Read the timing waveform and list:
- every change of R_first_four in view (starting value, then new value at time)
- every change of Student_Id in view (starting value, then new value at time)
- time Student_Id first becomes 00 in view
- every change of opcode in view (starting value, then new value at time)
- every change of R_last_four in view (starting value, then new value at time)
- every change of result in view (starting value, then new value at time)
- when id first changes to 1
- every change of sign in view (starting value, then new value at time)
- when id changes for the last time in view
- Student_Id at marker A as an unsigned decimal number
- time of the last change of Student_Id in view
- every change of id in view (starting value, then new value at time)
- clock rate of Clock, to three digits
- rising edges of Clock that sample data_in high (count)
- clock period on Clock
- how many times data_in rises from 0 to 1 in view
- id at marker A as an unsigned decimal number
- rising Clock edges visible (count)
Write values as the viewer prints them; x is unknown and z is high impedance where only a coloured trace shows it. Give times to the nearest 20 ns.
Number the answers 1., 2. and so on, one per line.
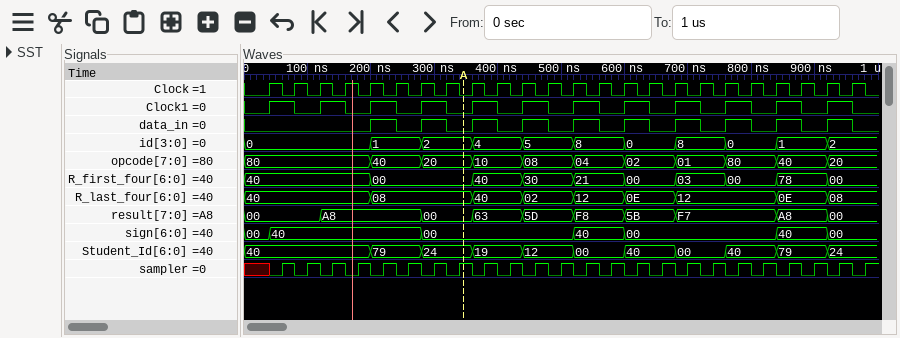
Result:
1. 40, 00 at 200 ns, 40 at 360 ns, 30 at 440 ns, 21 at 520 ns, 00 at 600 ns, 03 at 680 ns, 00 at 760 ns, 78 at 840 ns, 00 at 920 ns
2. 40, 79 at 200 ns, 24 at 280 ns, 19 at 360 ns, 12 at 440 ns, 00 at 520 ns, 40 at 600 ns, 00 at 680 ns, 40 at 760 ns, 79 at 840 ns, 24 at 920 ns
3. 520 ns
4. 80, 40 at 200 ns, 20 at 280 ns, 10 at 360 ns, 08 at 440 ns, 04 at 520 ns, 02 at 600 ns, 01 at 680 ns, 80 at 760 ns, 40 at 840 ns, 20 at 920 ns
5. 40, 08 at 200 ns, 40 at 360 ns, 02 at 440 ns, 12 at 520 ns, 0E at 600 ns, 12 at 680 ns, 0E at 840 ns, 08 at 920 ns
6. 00, A8 at 120 ns, 00 at 280 ns, 63 at 360 ns, 5D at 440 ns, F8 at 520 ns, 5B at 600 ns, F7 at 680 ns, A8 at 840 ns, 00 at 920 ns
7. 200 ns
8. 00, 40 at 40 ns, 00 at 280 ns, 40 at 520 ns, 00 at 600 ns, 40 at 840 ns, 00 at 920 ns
9. 920 ns
10. 36
11. 920 ns
12. 0, 1 at 200 ns, 2 at 280 ns, 4 at 360 ns, 5 at 440 ns, 8 at 520 ns, 0 at 600 ns, 8 at 680 ns, 0 at 760 ns, 1 at 840 ns, 2 at 920 ns
13. 25.0 MHz
14. 10
15. 40 ns
16. 10
17. 2
18. 24
